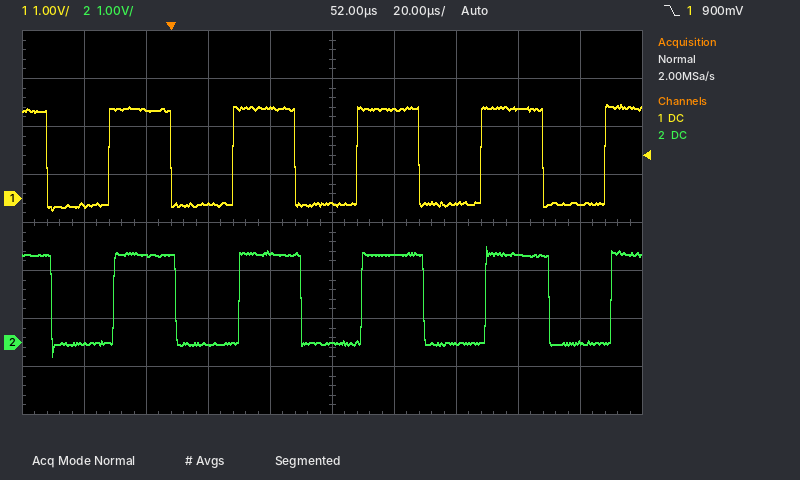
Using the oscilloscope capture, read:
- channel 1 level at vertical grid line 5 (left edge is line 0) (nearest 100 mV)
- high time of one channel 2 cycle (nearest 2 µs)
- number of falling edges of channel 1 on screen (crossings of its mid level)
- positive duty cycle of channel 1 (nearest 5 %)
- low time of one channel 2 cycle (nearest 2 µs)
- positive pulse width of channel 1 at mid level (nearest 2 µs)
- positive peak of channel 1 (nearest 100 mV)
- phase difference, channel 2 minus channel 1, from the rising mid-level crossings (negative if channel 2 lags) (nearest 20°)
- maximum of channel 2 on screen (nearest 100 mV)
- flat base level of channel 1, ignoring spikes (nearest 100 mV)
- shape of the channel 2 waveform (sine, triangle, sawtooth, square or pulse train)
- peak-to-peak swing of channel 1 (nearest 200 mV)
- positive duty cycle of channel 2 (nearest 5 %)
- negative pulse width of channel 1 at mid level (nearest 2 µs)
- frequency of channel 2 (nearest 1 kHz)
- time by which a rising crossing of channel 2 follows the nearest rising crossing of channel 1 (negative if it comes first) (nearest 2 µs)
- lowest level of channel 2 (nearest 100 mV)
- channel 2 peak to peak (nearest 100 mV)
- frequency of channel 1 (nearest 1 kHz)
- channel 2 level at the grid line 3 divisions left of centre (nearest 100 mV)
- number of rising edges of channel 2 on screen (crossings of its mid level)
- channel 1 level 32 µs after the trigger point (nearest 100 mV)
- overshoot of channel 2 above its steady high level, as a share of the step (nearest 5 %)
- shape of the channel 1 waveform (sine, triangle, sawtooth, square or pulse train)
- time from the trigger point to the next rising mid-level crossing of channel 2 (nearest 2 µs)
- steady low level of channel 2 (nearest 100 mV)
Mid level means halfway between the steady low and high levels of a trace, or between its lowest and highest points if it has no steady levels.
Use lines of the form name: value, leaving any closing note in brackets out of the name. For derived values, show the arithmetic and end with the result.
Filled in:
channel 1 level at vertical grid line 5 (left edge is line 0): -100 mV
high time of one channel 2 cycle: 20 µs
number of falling edges of channel 1 on screen: 5
positive duty cycle of channel 1: 20 µs / 40 µs ≈ 50 %
low time of one channel 2 cycle: 20 µs
positive pulse width of channel 1 at mid level: 20 µs
positive peak of channel 1: 2.0 V
phase difference, channel 2 minus channel 1, from the rising mid-level crossings (negative if channel 2 lags): −360° × (+2 µs) / 40 µs ≈ -18.0°, so -20° to the nearest 20°
maximum of channel 2 on screen: 2.0 V
flat base level of channel 1, ignoring spikes: -100 mV
shape of the channel 2 waveform: square
peak-to-peak swing of channel 1: 2.2 V
positive duty cycle of channel 2: 20 µs / 40 µs ≈ 50 %
negative pulse width of channel 1 at mid level: 20 µs
frequency of channel 2: 1 / 40 µs ≈ 25 kHz
time by which a rising crossing of channel 2 follows the nearest rising crossing of channel 1 (negative if it comes first): +2 µs
lowest level of channel 2: -300 mV
channel 2 peak to peak: 2.0 V − (-300 mV) = 2.3 V
frequency of channel 1: 1 / 40 µs ≈ 25 kHz
channel 2 level at the grid line 3 divisions left of centre: 1.8 V
number of rising edges of channel 2 on screen: 5
channel 1 level 32 µs after the trigger point: 1.9 V
overshoot of channel 2 above its steady high level, as a share of the step: 10 %
shape of the channel 1 waveform: square
time from the trigger point to the next rising mid-level crossing of channel 2: 22 µs
steady low level of channel 2: 0.0 V
